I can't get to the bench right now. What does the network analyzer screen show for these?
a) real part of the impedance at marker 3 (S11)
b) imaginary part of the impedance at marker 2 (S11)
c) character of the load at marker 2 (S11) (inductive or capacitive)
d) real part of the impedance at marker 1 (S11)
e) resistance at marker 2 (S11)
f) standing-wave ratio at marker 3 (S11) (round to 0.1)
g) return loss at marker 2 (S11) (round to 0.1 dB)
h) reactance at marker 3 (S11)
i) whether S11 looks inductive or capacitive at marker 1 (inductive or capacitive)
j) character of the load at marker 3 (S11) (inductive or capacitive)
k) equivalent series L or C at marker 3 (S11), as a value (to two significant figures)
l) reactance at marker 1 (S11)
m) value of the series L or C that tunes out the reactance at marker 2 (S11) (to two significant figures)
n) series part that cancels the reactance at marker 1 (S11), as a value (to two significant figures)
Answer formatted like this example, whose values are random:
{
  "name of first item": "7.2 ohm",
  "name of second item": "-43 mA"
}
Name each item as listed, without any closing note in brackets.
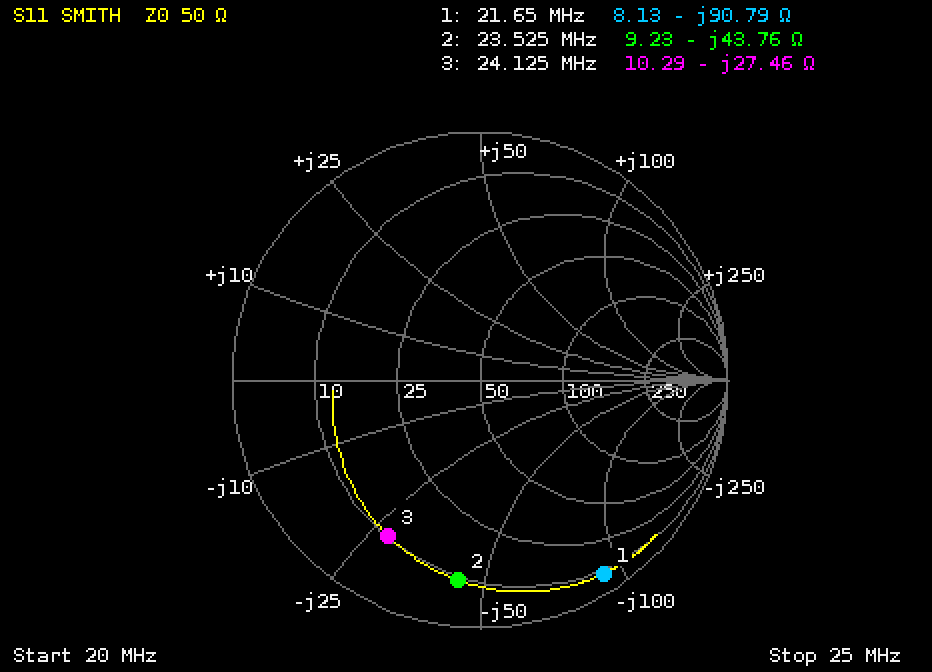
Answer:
{
  "real part of the impedance at marker 3": "10.29 Ω",
  "imaginary part of the impedance at marker 2": "-43.76 Ω",
  "character of the load at marker 2 (S11)": "capacitive",
  "real part of the impedance at marker 1": "8.13 Ω",
  "resistance at marker 2": "9.23 Ω",
  "standing-wave ratio at marker 3 (S11)": "6.4",
  "return loss at marker 2 (S11)": "1.8 dB",
  "reactance at marker 3": "-27.46 Ω",
  "whether S11 looks inductive or capacitive at marker 1": "capacitive",
  "character of the load at marker 3 (S11)": "capacitive",
  "equivalent series L or C at marker 3 (S11), as a value": "240 pF",
  "reactance at marker 1": "-90.79 Ω",
  "value of the series L or C that tunes out the reactance at marker 2 (S11)": "300 nH",
  "series part that cancels the reactance at marker 1 (S11), as a value": "670 nH"
}
